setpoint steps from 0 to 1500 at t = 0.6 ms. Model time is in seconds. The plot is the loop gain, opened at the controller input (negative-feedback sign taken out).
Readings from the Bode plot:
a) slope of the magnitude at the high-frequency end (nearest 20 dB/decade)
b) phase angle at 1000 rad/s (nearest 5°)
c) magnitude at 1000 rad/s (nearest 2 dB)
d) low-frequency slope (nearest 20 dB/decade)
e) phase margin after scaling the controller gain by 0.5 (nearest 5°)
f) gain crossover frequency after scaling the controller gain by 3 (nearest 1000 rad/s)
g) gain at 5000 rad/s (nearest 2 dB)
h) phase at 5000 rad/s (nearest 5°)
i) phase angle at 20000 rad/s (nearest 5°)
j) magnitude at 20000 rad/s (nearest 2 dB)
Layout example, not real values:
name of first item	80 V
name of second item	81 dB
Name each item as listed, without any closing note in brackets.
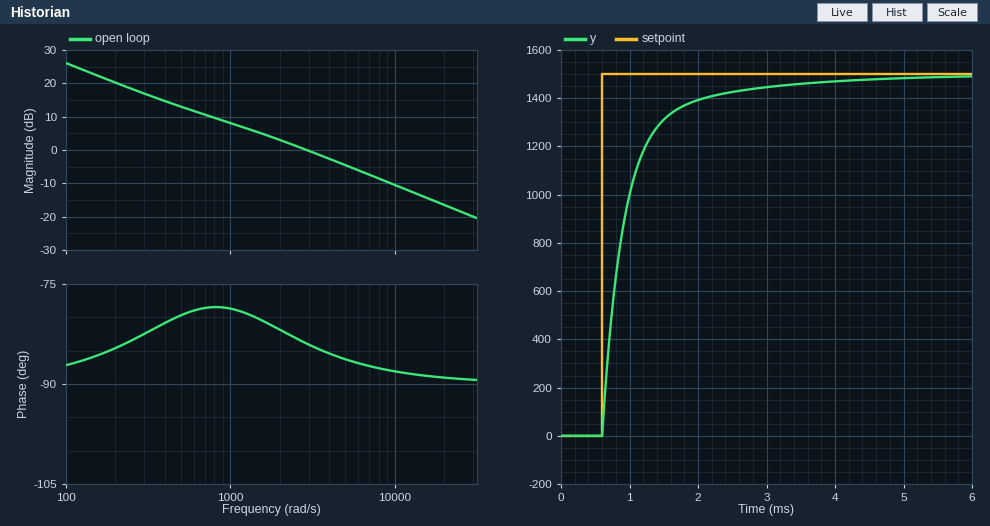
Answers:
slope of the magnitude at the high-frequency end	-20 dB/decade
phase angle at 1000 rad/s	-80°
magnitude at 1000 rad/s	8 dB
low-frequency slope	-20 dB/decade
phase margin after scaling the controller gain by 0.5	100°
gain crossover frequency after scaling the controller gain by 3	9000 rad/s
gain at 5000 rad/s	-4 dB
phase at 5000 rad/s	-85°
phase angle at 20000 rad/s	-90°
magnitude at 20000 rad/s	-16 dB
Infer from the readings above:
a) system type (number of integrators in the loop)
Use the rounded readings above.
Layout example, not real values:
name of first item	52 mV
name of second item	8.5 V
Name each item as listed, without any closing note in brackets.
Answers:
system type	1
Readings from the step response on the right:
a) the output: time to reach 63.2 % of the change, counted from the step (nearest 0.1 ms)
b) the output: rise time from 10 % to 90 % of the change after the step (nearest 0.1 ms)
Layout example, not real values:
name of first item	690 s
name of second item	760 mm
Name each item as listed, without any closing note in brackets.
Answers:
the output: time to reach 63.2 % of the change, counted from the step	0.4 ms
the output: rise time from 10 % to 90 % of the change after the step	1.0 ms
